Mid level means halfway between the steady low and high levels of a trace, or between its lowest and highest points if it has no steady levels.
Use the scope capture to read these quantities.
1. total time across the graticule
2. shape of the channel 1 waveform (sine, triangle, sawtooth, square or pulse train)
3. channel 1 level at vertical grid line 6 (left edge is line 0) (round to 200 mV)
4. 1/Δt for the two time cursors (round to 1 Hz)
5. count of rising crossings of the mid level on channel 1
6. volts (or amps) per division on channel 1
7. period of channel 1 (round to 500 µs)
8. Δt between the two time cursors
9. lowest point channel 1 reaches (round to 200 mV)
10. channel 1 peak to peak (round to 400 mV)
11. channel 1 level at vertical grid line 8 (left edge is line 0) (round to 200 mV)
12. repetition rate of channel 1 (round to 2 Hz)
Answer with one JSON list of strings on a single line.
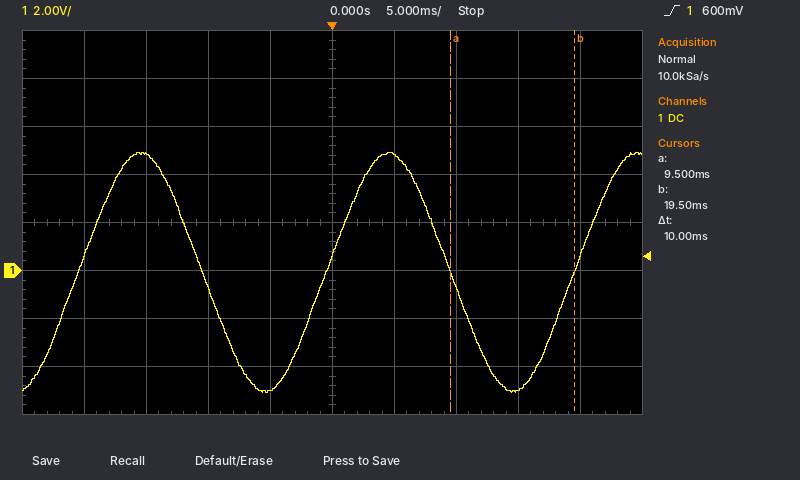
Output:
["50 ms", "sine", "4.8 V", "100 Hz", "3", "2 V", "20.0 ms", "10 ms", "-5.0 V", "10.0 V", "-5.0 V", "50 Hz"]
